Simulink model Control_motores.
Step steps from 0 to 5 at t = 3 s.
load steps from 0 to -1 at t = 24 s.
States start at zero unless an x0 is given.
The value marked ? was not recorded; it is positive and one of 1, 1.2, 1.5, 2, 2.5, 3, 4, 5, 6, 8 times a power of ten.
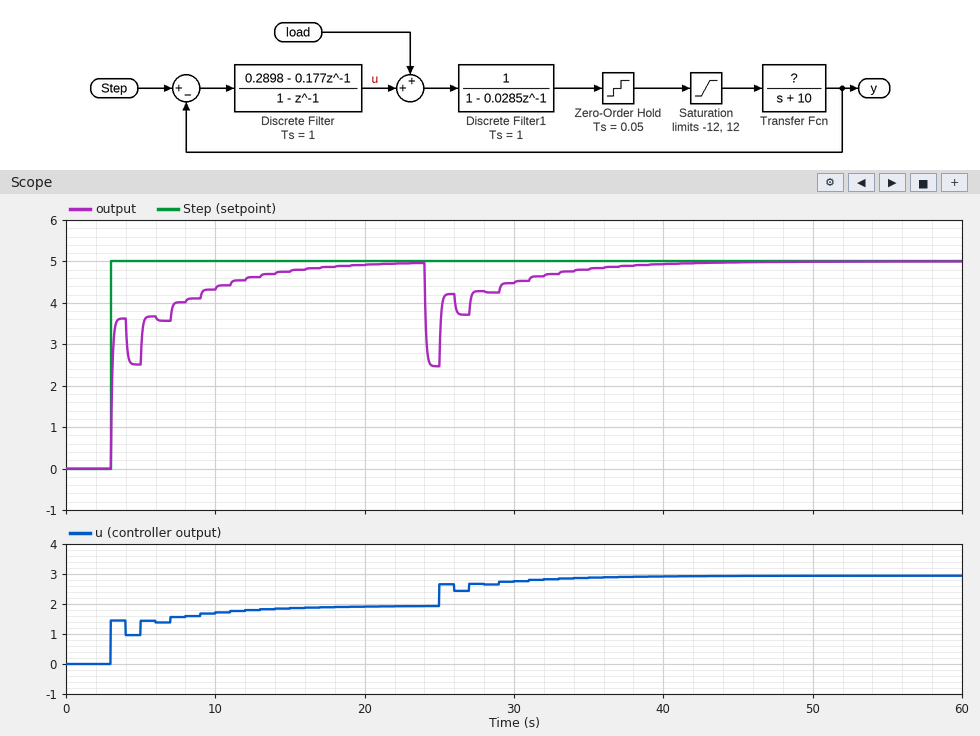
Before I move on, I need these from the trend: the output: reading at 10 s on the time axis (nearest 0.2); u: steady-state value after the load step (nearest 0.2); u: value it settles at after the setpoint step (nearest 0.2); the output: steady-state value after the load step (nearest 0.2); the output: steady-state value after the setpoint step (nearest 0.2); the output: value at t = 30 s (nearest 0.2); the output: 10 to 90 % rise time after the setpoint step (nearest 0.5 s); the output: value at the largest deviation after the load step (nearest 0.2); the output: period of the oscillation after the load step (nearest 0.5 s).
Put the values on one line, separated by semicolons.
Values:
4.4; 3.0; 2.0; 5.0; 5.0; 4.4; 8.0 s; 2.4; 2.0 s
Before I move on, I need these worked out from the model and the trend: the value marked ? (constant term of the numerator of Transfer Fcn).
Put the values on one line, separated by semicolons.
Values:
25
